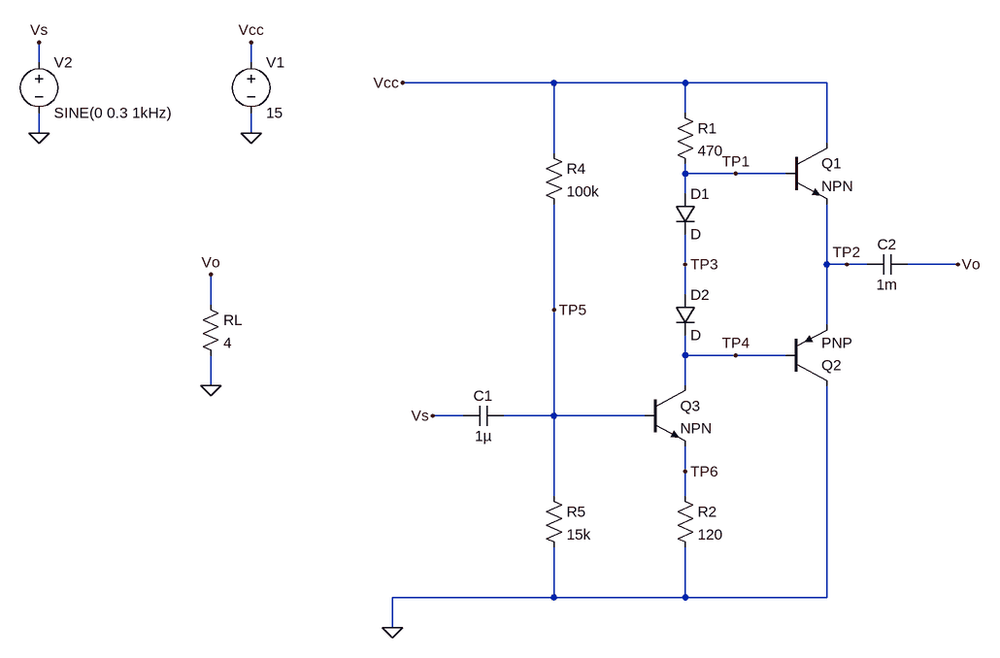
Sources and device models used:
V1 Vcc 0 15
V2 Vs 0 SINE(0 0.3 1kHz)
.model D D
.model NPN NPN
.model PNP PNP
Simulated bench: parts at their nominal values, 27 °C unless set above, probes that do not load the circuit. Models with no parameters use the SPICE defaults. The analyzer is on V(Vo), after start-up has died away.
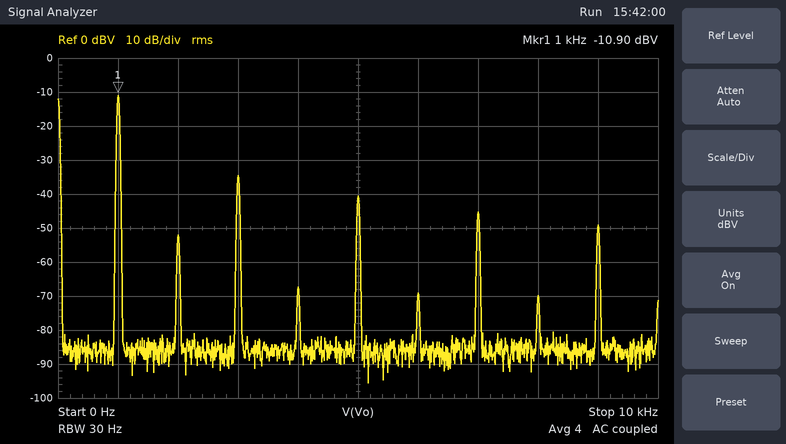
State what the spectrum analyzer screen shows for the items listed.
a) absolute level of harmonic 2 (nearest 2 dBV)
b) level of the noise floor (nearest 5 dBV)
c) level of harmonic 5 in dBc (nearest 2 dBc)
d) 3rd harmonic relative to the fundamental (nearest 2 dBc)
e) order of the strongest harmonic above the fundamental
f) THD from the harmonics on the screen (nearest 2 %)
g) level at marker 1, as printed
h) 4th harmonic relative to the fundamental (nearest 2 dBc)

-52 dBV
-85 dBV
-30 dBc
-24 dBc
3
8 %
-10.90 dBV
-56 dBc
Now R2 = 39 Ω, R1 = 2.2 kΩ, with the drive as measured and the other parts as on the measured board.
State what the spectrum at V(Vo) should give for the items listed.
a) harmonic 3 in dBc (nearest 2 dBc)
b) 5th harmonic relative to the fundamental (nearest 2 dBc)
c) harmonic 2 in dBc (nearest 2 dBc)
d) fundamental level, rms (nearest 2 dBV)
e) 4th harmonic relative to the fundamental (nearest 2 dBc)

-26 dBc
-38 dBc
-20 dBc
2 dBV
-42 dBc
